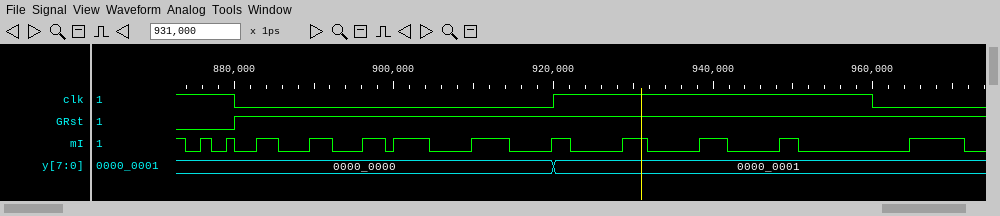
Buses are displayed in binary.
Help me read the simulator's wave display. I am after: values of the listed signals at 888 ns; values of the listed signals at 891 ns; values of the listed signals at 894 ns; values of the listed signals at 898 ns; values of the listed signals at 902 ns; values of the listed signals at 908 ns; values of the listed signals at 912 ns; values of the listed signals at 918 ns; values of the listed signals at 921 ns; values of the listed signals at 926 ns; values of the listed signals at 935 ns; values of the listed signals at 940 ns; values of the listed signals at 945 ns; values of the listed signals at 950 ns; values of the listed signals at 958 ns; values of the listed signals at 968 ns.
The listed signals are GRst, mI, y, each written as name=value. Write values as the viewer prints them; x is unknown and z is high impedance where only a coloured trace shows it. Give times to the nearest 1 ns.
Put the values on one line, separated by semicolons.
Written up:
GRst=1, mI=0, y=0000_0000; GRst=1, mI=1, y=0000_0000; GRst=1, mI=0, y=0000_0000; GRst=1, mI=1, y=0000_0000; GRst=1, mI=1, y=0000_0000; GRst=1, mI=0, y=0000_0000; GRst=1, mI=1, y=0000_0000; GRst=1, mI=0, y=0000_0000; GRst=1, mI=1, y=0000_0001; GRst=1, mI=0, y=0000_0001; GRst=1, mI=0, y=0000_0001; GRst=1, mI=1, y=0000_0001; GRst=1, mI=0, y=0000_0001; GRst=1, mI=1, y=0000_0001; GRst=1, mI=0, y=0000_0001; GRst=1, mI=1, y=0000_0001
